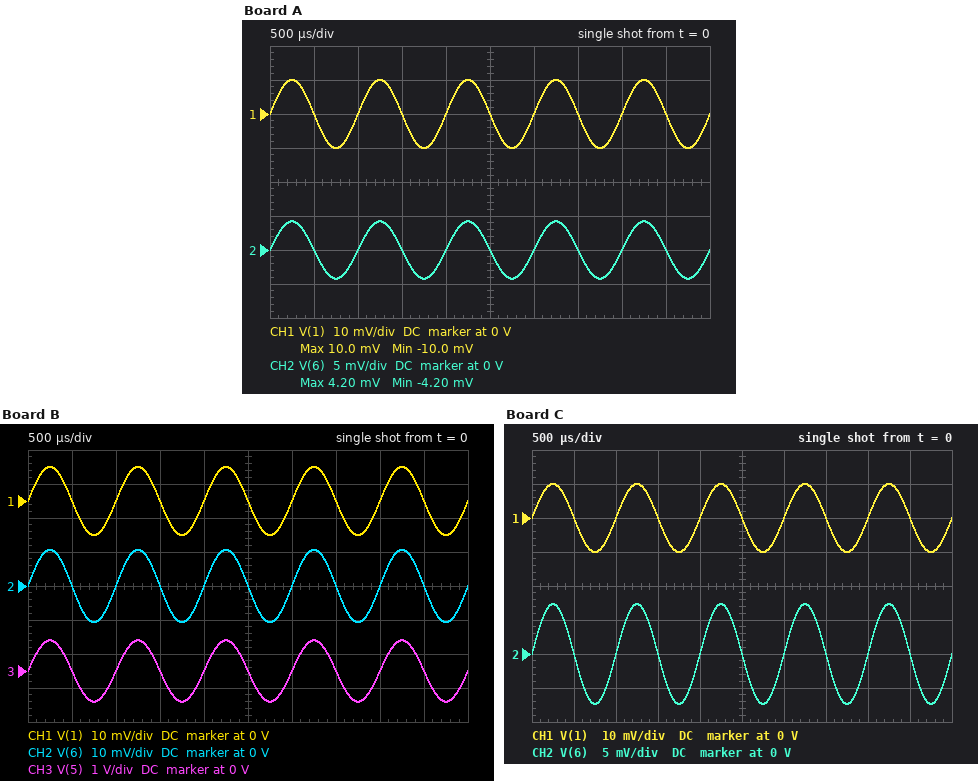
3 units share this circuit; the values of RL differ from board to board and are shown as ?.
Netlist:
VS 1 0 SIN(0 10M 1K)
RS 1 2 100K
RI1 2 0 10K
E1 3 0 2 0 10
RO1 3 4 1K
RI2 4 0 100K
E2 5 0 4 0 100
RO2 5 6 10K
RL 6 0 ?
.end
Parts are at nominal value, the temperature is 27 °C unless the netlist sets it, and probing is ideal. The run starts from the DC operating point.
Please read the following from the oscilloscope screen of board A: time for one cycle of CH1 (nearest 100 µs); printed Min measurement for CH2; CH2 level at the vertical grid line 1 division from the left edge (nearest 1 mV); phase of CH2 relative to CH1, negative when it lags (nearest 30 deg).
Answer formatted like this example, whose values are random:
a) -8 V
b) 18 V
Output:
a) 1.0 ms
b) -4.20 mV
c) 0 V
d) 0 deg
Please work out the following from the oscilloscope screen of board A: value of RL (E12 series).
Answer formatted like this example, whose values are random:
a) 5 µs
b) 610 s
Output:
a) 47 Ω
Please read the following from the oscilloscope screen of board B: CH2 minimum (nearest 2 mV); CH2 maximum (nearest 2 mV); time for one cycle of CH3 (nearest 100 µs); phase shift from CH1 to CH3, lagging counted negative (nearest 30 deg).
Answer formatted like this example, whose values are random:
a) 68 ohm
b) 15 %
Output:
a) -10 mV
b) 10 mV
c) 1.0 ms
d) 0 deg
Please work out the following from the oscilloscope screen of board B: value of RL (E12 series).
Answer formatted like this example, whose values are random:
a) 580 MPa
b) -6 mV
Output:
a) 120 Ω
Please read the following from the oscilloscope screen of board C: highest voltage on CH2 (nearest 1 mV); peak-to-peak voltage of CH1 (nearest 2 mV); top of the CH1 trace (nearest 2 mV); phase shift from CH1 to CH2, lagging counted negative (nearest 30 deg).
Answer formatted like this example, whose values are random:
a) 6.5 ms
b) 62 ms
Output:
a) 7 mV
b) 20 mV
c) 10 mV
d) 0 deg
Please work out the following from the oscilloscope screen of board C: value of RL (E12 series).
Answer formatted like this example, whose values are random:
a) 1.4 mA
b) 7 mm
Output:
a) 82 Ω
